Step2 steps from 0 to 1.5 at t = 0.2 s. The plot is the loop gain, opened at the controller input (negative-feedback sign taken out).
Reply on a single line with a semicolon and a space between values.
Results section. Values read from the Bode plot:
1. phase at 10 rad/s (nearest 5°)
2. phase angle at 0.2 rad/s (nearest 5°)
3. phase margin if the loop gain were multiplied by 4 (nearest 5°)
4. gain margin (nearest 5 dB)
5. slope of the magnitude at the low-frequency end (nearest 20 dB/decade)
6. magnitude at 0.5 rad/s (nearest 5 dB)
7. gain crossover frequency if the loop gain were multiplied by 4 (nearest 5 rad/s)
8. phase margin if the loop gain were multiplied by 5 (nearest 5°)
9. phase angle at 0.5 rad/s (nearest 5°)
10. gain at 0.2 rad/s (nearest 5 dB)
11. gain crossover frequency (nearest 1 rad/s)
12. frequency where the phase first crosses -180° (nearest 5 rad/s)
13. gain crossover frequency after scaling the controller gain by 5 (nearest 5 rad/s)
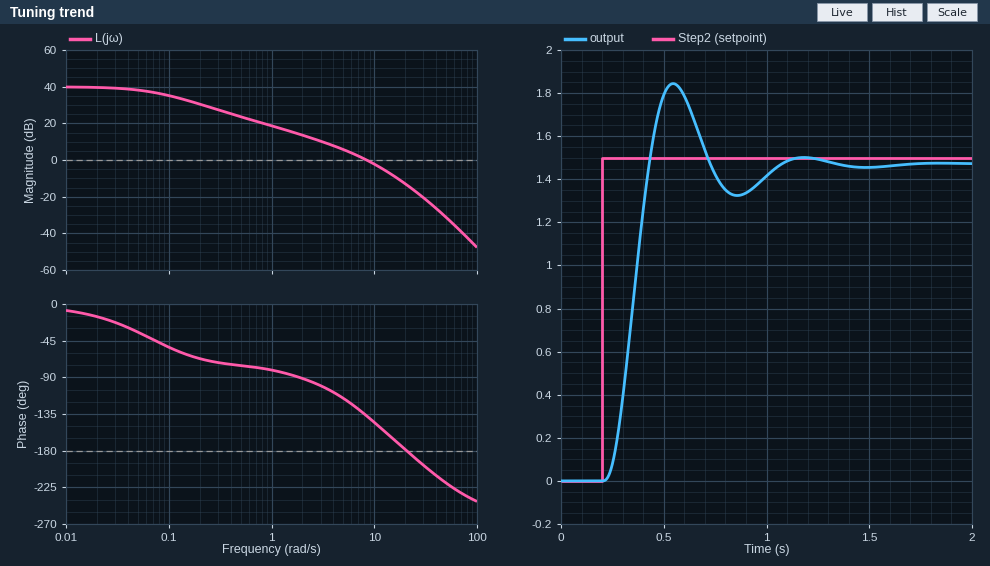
-145°; -65°; 5°; 15 dB; 0 dB/decade; 25 dB; 20 rad/s; 0°; -75°; 30 dB; 8 rad/s; 20 rad/s; 20 rad/s
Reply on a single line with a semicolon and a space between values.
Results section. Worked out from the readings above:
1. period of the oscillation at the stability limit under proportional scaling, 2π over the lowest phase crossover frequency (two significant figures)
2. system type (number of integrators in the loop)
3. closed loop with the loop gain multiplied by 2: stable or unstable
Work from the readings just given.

0.31 s; 0; stable
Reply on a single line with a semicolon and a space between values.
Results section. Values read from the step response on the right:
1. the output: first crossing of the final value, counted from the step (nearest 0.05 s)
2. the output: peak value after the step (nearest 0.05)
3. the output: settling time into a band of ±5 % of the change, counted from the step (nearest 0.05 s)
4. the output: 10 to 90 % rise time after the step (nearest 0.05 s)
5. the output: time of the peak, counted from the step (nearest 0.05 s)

0.25 s; 1.85; 0.80 s; 0.15 s; 0.35 s
